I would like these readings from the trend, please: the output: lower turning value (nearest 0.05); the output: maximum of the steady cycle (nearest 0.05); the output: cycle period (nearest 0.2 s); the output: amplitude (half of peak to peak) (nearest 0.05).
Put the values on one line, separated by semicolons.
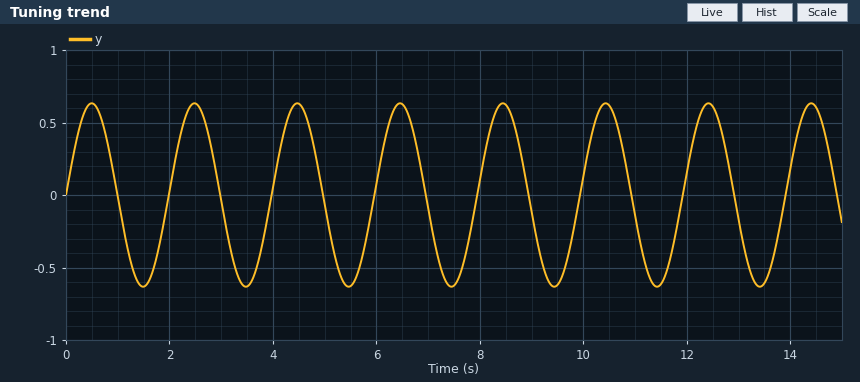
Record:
-0.65; 0.65; 2.0 s; 0.65
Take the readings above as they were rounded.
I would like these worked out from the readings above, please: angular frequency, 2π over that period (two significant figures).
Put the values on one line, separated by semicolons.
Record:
3.1 rad/s
